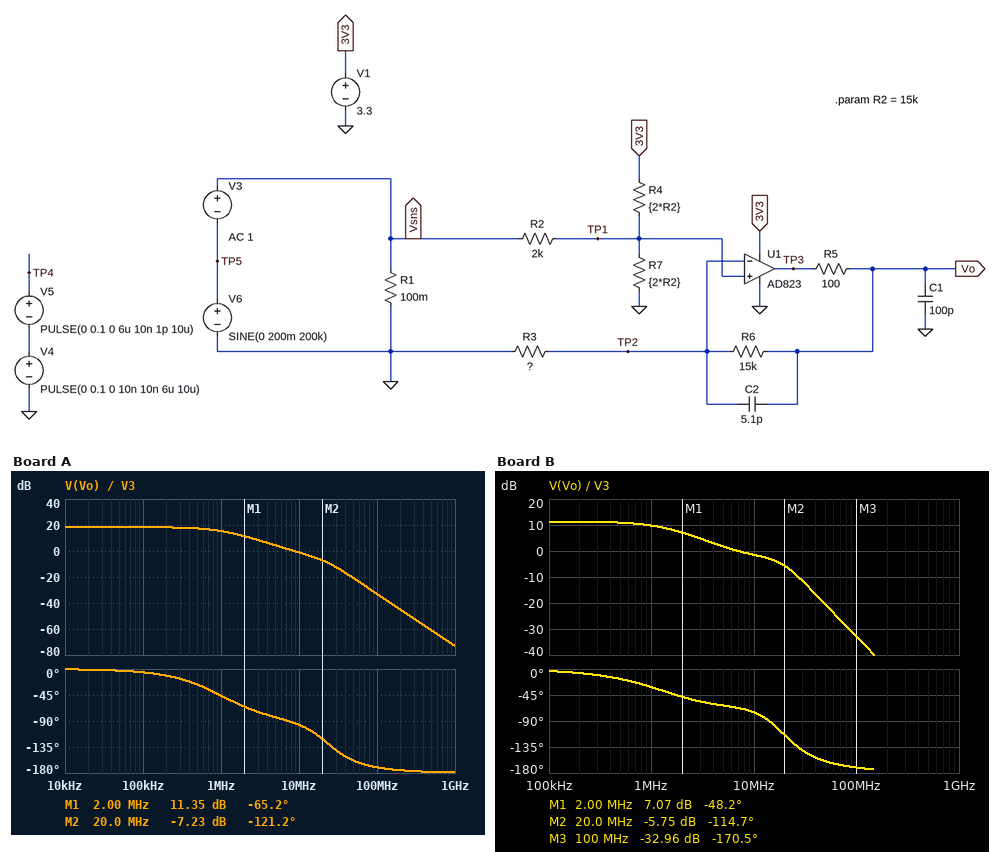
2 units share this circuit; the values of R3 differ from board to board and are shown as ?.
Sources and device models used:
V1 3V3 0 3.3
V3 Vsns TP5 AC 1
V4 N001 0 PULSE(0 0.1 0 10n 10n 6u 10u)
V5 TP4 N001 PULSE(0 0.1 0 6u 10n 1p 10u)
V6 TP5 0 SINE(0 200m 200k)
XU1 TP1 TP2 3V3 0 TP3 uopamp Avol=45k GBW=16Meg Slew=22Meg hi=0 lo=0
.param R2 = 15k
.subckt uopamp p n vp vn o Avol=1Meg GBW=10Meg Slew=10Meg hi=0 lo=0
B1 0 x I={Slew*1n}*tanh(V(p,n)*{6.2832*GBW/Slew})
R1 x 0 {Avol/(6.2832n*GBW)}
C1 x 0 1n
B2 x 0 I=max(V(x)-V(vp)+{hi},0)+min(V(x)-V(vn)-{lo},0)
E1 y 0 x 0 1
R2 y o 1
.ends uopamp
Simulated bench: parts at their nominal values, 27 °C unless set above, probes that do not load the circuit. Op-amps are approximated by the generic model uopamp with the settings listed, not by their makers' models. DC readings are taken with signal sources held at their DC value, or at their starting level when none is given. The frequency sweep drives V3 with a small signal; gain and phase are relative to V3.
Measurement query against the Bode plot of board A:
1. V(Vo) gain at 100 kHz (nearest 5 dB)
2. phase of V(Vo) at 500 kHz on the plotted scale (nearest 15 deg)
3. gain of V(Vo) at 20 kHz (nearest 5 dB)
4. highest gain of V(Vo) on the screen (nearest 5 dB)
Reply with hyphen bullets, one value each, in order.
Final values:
- 20 dB
- -30 deg
- 20 dB
- 20 dB
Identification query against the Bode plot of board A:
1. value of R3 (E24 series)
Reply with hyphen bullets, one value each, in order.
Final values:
- 1.8 kΩ
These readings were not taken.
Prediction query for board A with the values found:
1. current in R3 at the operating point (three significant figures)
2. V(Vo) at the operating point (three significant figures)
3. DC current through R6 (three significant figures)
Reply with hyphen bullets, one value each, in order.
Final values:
- 108 µA
- 1.81 V
- 108 µA
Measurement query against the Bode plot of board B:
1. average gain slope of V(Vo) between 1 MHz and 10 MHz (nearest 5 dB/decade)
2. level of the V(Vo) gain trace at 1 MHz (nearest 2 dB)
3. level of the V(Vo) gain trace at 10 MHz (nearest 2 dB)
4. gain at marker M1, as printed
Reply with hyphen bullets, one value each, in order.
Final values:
- -10 dB/decade
- 10 dB
- -2 dB
- 7.07 dB
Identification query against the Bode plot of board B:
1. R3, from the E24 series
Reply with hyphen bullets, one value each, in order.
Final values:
- 4.7 kΩ
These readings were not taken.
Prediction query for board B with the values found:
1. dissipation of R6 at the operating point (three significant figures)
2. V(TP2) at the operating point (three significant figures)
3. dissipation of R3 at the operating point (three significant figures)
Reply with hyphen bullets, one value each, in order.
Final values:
- 25.6 µW
- 194 mV
- 8.02 µW
